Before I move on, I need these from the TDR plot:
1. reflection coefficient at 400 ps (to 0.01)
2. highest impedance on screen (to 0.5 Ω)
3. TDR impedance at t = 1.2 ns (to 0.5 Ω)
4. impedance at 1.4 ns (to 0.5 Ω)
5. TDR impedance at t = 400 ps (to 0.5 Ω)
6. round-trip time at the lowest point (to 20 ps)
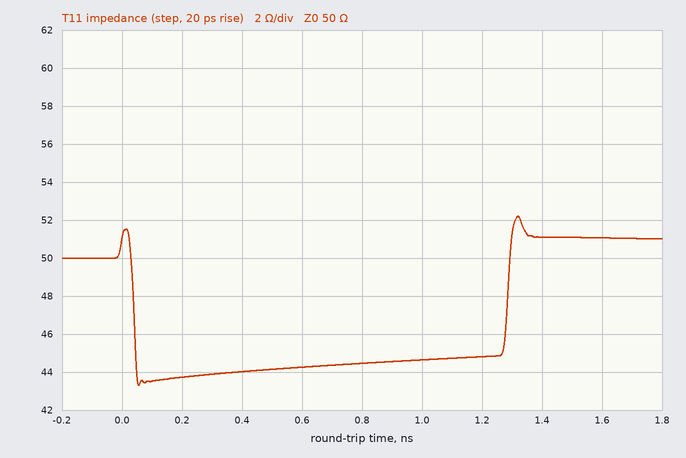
-0.06
52.0 Ω
45.0 Ω
51.0 Ω
44.0 Ω
60 ps
